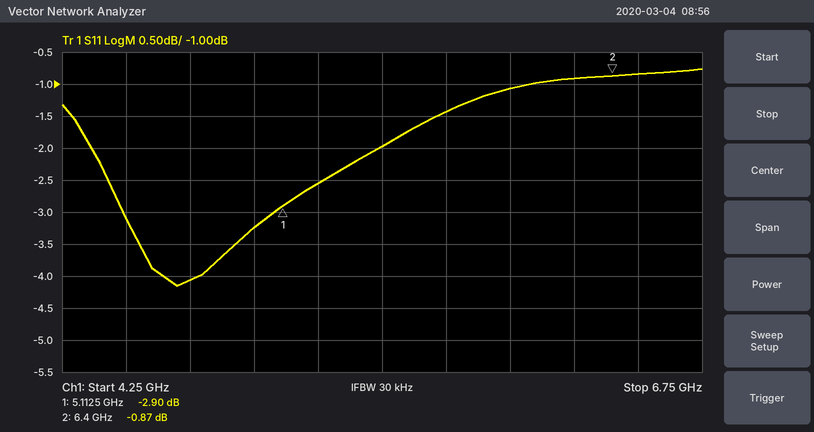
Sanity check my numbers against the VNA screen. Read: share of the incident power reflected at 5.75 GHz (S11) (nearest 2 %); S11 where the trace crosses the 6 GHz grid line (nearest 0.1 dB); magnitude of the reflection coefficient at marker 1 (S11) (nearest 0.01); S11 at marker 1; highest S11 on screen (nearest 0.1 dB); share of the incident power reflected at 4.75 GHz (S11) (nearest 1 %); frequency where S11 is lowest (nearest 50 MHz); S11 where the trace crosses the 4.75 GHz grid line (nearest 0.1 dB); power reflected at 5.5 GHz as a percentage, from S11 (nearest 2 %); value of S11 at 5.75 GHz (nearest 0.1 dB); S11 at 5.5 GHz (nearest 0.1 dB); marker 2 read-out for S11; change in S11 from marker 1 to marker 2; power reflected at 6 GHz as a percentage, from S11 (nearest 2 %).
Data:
72 %
-1.1 dB
0.72
-2.90 dB
-0.8 dB
39 %
4.70 GHz
-4.1 dB
64 %
-1.4 dB
-2.0 dB
-0.87 dB
2.03 dB
78 %
